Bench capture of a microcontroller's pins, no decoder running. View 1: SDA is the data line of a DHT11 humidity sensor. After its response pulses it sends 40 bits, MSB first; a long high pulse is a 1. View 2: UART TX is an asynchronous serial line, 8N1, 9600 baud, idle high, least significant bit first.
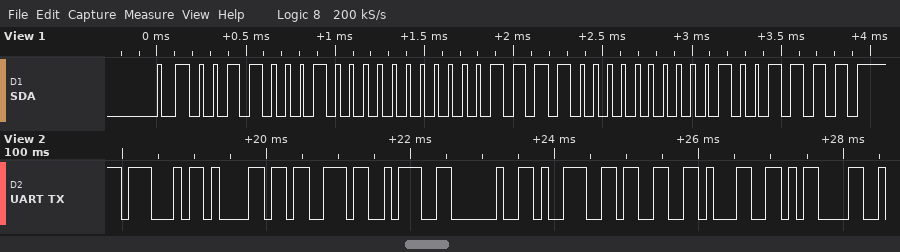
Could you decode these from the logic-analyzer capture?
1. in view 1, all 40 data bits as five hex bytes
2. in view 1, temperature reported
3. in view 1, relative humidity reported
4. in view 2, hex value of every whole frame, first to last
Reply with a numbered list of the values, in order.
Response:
1. 31 00 1E 00 4F
2. 30.0 °C
3. 49 %
4. 0x47 0x61 0x73 0x3A 0x20 0x39 0x33 0x31 0x0D
